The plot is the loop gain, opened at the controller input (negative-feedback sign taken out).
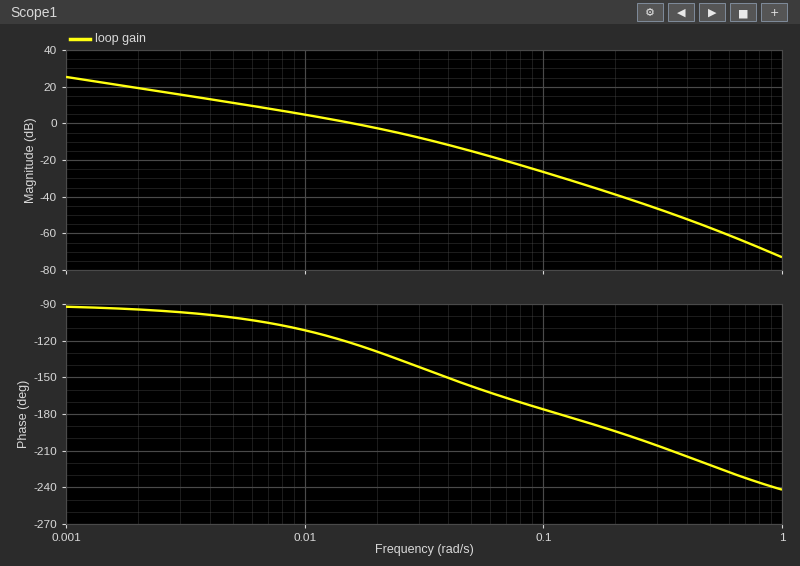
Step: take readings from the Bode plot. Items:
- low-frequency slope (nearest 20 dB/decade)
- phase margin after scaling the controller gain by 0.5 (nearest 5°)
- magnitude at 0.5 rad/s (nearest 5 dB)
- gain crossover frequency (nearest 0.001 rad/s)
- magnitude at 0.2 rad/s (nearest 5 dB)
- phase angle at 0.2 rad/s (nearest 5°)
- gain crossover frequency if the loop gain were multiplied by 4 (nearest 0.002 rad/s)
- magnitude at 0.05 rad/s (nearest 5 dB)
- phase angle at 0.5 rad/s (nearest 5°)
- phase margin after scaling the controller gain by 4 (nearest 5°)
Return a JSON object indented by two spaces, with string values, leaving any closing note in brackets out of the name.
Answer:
{
  "low-frequency slope": "-20 dB/decade",
  "phase margin after scaling the controller gain by 0.5": "70°",
  "magnitude at 0.5 rad/s": "-55 dB",
  "gain crossover frequency": "0.016 rad/s",
  "magnitude at 0.2 rad/s": "-40 dB",
  "phase angle at 0.2 rad/s": "-195°",
  "gain crossover frequency if the loop gain were multiplied by 4": "0.040 rad/s",
  "magnitude at 0.05 rad/s": "-15 dB",
  "phase angle at 0.5 rad/s": "-220°",
  "phase margin after scaling the controller gain by 4": "30°"
}
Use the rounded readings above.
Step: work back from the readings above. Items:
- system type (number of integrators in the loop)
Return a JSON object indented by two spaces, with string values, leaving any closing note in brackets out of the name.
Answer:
{
  "system type": "1"
}
